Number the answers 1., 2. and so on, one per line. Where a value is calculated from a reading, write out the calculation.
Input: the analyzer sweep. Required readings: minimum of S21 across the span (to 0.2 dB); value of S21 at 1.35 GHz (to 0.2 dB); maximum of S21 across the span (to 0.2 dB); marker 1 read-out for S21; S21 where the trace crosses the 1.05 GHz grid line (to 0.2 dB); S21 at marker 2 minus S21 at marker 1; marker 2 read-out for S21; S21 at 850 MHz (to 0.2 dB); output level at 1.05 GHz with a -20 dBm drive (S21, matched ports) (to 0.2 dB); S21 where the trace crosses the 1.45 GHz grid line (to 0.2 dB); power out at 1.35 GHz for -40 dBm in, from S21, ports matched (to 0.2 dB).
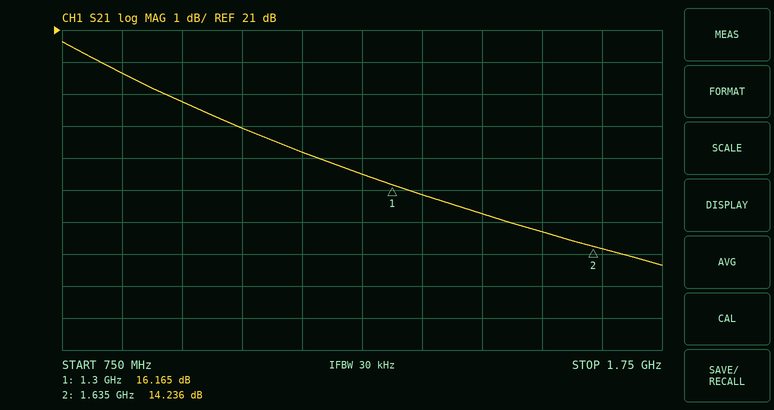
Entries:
1. 13.6 dB
2. 15.8 dB
3. 20.6 dB
4. 16.165 dB
5. 18.0 dB
6. 14.236 − (16.165) = -1.929 dB
7. 14.236 dB
8. 19.6 dB
9. -20 dBm + (18.0 dB) = -2.0 dBm
10. 15.2 dB
11. -40 dBm + (15.8 dB) = -24.2 dBm
